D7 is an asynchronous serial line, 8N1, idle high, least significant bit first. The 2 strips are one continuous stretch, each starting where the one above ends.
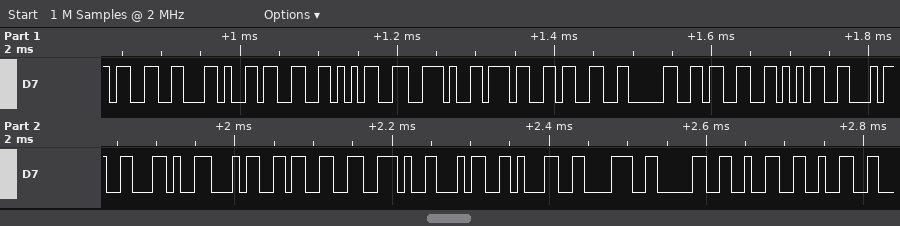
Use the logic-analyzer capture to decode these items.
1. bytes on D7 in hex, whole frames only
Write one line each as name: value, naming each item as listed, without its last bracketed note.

bytes on D7 in hex, whole frames only: 33 2C 33 35 2E 37 33 30 33 35 34 2C 34 33 2E 34 31 38 30 32 32
